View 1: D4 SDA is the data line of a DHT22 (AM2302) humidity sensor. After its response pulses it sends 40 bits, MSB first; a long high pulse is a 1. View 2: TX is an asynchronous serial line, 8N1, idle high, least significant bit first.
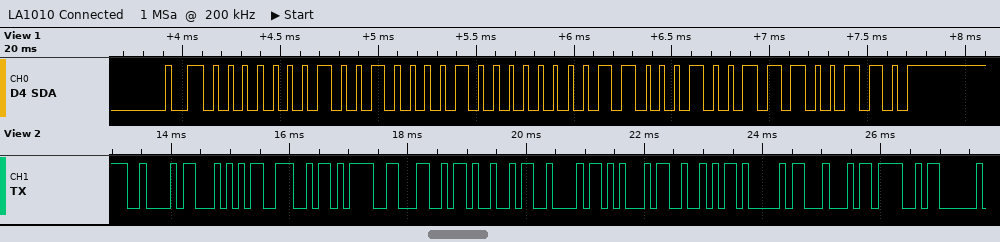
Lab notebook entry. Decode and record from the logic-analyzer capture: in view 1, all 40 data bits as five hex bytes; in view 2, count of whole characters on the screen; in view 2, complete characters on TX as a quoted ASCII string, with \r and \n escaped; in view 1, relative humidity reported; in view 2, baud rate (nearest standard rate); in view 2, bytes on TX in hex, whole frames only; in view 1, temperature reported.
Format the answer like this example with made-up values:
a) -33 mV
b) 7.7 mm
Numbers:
a) 01 21 00 C4 E6
b) 12
c) "BTN=LIBERADO"
d) 28.9 %
e) 9600 baud
f) 0x42 0x54 0x4E 0x3D 0x4C 0x49 0x42 0x45 0x52 0x41 0x44 0x4F
g) 19.6 °C
